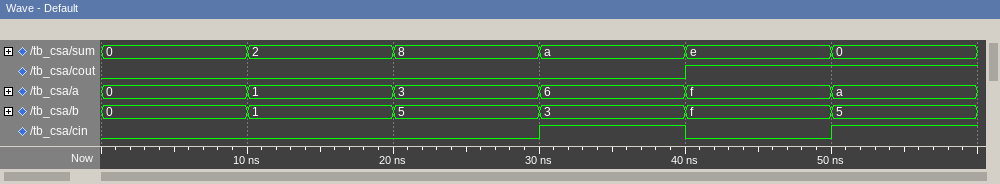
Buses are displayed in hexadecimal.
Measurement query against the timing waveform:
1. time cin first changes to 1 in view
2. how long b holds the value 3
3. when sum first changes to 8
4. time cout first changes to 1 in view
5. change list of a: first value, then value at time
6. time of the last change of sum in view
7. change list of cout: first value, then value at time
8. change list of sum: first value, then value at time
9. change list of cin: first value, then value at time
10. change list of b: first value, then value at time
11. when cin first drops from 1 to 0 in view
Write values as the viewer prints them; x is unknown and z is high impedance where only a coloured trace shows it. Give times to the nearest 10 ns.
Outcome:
30 ns
10 ns
20 ns
40 ns
0, 1 at 10 ns, 3 at 20 ns, 6 at 30 ns, f at 40 ns, a at 50 ns
50 ns
0, 1 at 40 ns
0, 2 at 10 ns, 8 at 20 ns, a at 30 ns, e at 40 ns, 0 at 50 ns
0, 1 at 30 ns, 0 at 40 ns, 1 at 50 ns
0, 1 at 10 ns, 5 at 20 ns, 3 at 30 ns, f at 40 ns, 5 at 50 ns
40 ns
